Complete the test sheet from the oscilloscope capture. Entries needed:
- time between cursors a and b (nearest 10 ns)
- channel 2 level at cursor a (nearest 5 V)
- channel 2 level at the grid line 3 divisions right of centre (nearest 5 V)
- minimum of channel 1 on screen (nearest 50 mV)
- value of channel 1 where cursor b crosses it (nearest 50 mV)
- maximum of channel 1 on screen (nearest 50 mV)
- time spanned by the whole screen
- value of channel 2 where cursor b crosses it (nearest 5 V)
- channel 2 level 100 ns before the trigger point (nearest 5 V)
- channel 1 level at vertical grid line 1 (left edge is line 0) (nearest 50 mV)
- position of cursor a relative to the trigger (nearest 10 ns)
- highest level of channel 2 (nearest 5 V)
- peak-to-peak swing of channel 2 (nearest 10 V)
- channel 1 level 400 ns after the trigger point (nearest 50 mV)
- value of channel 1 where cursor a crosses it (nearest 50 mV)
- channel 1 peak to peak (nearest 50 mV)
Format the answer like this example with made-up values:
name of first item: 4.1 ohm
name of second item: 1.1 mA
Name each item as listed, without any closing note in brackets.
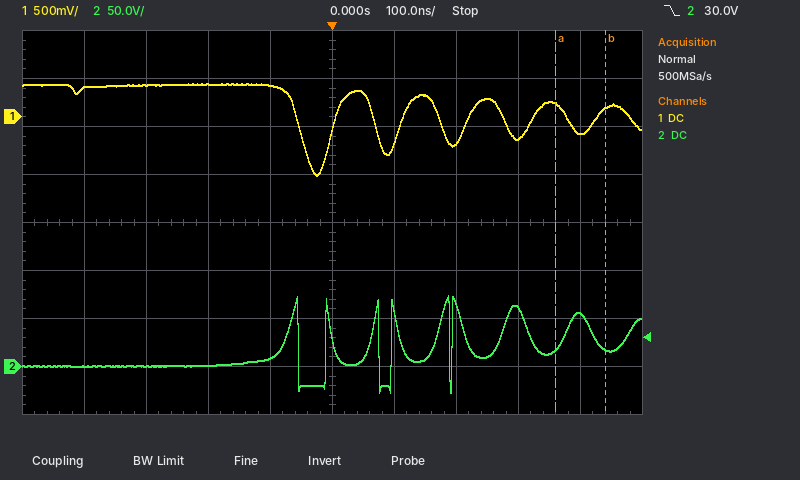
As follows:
time between cursors a and b: 80 ns
channel 2 level at cursor a: 20 V
channel 2 level at the grid line 3 divisions right of centre: 60 V
minimum of channel 1 on screen: -600 mV
value of channel 1 where cursor b crosses it: 100 mV
maximum of channel 1 on screen: 350 mV
time spanned by the whole screen: 1 µs
value of channel 2 where cursor b crosses it: 20 V
channel 2 level 100 ns before the trigger point: 10 V
channel 1 level at vertical grid line 1 (left edge is line 0): 300 mV
position of cursor a relative to the trigger: +360 ns
highest level of channel 2: 75 V
peak-to-peak swing of channel 2: 100 V
channel 1 level 400 ns after the trigger point: -150 mV
value of channel 1 where cursor a crosses it: 150 mV
channel 1 peak to peak: 950 mV
